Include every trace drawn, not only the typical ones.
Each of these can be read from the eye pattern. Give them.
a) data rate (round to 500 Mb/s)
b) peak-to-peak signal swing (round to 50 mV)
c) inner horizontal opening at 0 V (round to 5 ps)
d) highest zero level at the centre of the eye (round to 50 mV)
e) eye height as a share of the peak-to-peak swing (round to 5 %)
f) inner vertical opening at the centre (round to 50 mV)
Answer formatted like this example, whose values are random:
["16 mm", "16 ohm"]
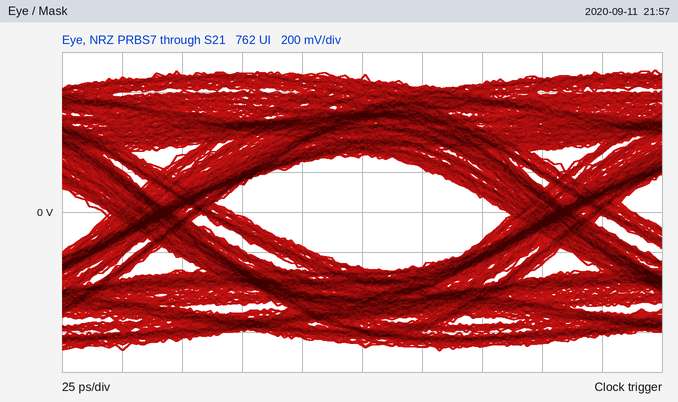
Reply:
["6.0 Gb/s", "1.40 V", "115 ps", "-300 mV", "40 %", "550 mV"]
